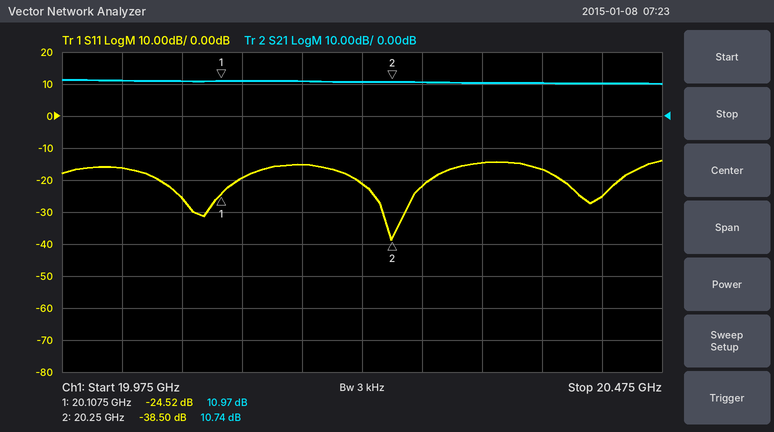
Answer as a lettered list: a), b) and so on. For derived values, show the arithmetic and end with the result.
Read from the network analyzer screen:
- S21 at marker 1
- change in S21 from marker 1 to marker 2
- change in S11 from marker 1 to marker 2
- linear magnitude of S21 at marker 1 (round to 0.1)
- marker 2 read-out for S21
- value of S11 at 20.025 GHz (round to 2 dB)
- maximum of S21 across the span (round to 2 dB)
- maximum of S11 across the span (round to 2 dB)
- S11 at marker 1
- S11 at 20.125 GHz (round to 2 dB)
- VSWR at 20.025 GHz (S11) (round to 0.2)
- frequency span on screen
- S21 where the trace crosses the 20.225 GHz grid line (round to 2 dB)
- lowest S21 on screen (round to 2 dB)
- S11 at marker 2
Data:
a) 10.97 dB
b) 10.74 − (10.97) = -0.23 dB
c) -38.5 − (-24.52) = -13.98 dB
d) 10^(10.97/20) ≈ 3.5
e) 10.74 dB
f) -16 dB
g) 12 dB
h) -14 dB
i) -24.52 dB
j) -20 dB
k) |Γ| = 10^(-16/20) = 0.1585; VSWR = (1 + 0.1585)/(1 − 0.1585) ≈ 1.4
l) 500 MHz
m) 10 dB
n) 10 dB
o) -38.50 dB
